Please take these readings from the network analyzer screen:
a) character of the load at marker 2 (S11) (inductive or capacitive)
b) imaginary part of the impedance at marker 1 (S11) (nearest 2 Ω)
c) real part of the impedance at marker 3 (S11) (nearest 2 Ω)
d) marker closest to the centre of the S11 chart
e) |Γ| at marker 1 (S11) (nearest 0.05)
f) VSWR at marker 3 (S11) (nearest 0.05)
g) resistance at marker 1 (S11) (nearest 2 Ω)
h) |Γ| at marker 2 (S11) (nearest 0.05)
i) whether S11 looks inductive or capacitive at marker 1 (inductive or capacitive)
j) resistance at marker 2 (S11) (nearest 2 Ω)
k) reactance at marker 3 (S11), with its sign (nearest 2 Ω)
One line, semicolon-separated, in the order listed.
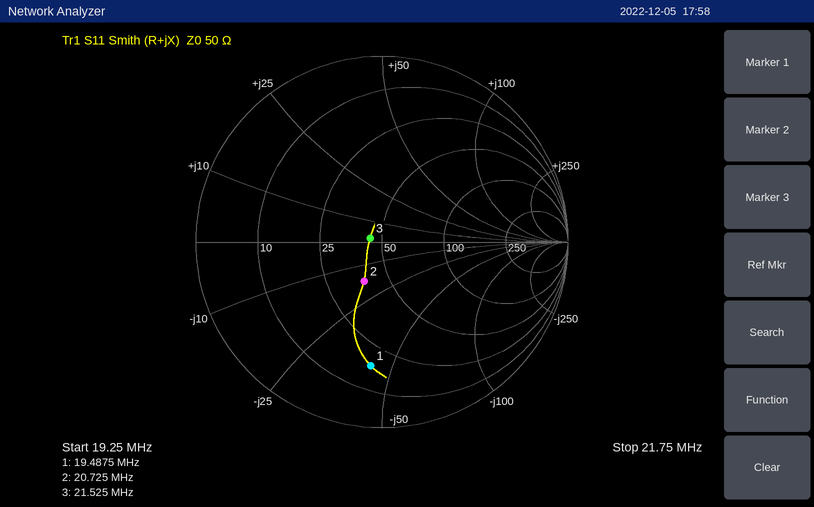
capacitive; -42 Ω; 44 Ω; marker 3; 0.65; 1.15; 18 Ω; 0.25; capacitive; 38 Ω; +2 Ω
